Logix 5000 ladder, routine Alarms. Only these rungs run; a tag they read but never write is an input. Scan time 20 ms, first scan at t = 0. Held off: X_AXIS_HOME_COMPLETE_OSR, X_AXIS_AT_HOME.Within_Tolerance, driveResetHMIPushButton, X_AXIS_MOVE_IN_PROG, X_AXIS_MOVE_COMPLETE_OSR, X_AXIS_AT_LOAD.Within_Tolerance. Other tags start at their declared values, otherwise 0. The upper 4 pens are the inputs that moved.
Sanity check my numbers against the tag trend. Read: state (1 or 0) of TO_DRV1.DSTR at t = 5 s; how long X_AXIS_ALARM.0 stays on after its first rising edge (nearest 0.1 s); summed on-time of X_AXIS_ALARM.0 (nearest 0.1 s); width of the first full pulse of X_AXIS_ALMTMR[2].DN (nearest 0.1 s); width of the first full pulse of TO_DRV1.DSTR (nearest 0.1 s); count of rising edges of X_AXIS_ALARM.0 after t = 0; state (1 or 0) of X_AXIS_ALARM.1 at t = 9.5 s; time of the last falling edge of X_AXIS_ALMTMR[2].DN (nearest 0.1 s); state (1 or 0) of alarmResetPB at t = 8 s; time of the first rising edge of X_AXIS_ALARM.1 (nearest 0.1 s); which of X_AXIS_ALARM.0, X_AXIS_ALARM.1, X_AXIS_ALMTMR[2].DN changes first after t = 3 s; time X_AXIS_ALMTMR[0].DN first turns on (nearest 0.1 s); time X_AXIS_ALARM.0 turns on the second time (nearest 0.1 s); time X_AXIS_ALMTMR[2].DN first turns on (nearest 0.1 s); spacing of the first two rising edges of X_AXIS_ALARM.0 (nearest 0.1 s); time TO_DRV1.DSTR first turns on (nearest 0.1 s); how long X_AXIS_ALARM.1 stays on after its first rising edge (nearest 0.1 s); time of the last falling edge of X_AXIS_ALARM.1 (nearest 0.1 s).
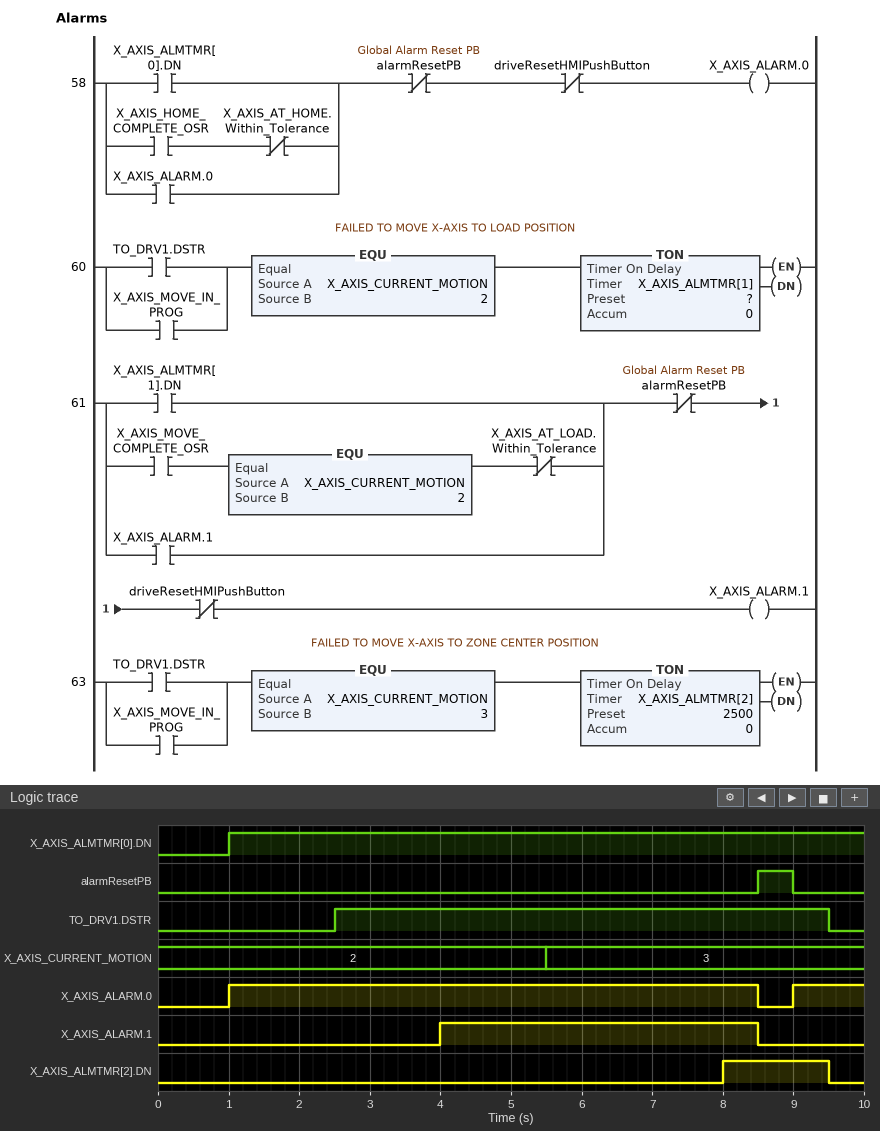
1
7.5 s
8.5 s
1.5 s
7.0 s
2
0
9.5 s
0
4.0 s
X_AXIS_ALARM.1
1.0 s
9.0 s
8.0 s
8.0 s
2.5 s
4.5 s
8.5 s
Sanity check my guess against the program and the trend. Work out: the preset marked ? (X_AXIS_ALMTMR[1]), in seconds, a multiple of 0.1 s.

1.5 s
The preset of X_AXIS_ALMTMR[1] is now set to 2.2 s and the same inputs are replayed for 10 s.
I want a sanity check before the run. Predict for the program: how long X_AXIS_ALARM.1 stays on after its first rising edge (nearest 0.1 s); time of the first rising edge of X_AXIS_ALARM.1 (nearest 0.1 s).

3.8 s
4.7 s
